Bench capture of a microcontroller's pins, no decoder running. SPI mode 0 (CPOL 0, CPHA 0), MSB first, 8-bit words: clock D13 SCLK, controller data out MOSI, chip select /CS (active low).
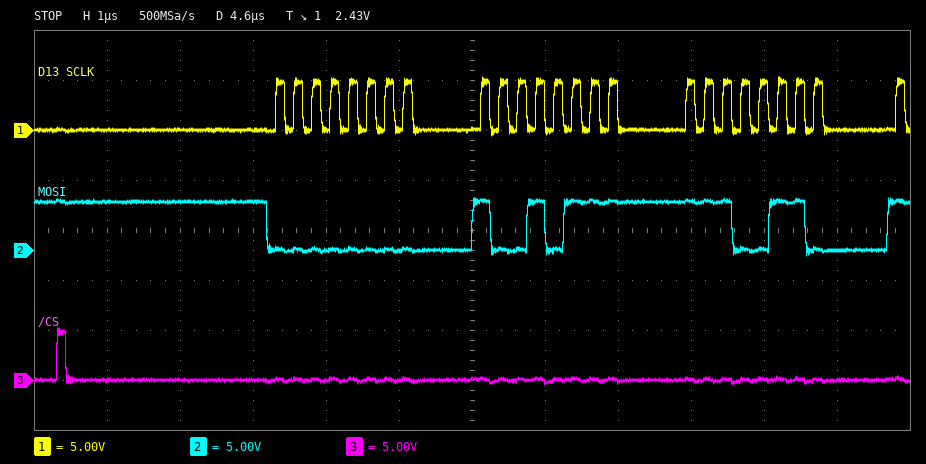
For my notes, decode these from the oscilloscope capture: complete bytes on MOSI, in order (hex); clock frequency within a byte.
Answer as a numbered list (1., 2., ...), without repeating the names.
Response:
1. 0x00 0x97 0xE6
2. 4 MHz
